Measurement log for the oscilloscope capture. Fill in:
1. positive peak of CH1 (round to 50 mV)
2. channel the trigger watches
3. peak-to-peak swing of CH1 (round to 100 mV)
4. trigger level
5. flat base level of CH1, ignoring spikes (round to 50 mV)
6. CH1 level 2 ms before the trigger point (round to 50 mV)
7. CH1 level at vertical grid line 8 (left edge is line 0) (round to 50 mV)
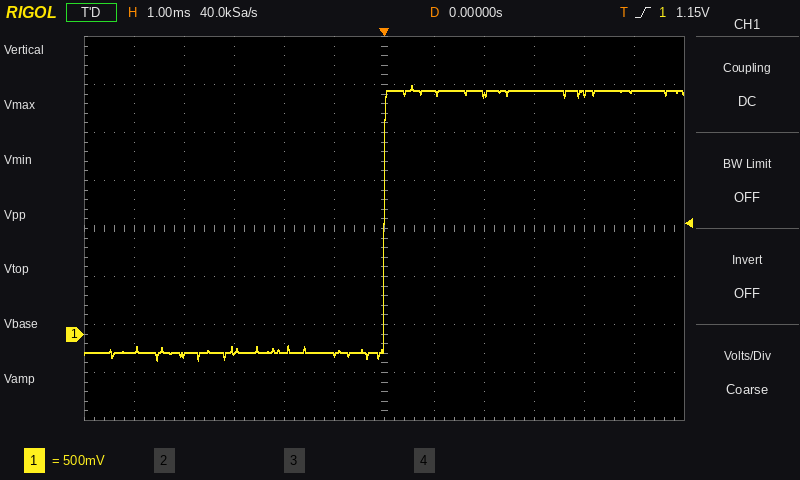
2.60 V
CH1
2.90 V
1.15 V
-200 mV
-200 mV
2.50 V
